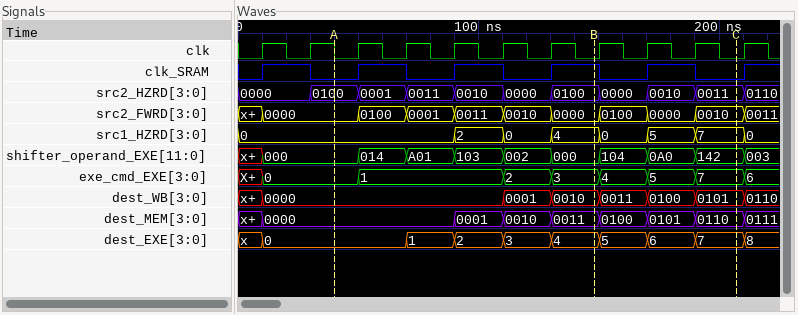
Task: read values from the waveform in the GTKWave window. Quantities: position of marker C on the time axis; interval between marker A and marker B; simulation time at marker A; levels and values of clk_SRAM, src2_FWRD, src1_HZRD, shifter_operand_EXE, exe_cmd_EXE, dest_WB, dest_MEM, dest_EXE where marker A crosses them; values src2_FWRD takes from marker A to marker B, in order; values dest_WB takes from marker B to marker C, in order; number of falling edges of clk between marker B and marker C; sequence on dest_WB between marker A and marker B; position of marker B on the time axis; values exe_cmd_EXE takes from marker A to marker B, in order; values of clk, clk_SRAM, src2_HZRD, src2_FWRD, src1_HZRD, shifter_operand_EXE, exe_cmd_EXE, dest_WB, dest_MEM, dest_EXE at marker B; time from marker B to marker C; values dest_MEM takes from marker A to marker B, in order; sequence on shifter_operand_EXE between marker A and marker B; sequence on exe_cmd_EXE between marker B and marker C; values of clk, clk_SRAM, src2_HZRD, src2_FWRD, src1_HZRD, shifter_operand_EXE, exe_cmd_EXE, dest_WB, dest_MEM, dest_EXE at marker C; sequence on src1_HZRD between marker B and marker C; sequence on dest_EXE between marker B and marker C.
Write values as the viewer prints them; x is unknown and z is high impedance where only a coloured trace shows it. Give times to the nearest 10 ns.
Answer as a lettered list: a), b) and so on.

a) 210 ns
b) 110 ns
c) 40 ns
d) clk_SRAM=0, src2_FWRD=0000, src1_HZRD=0, shifter_operand_EXE=000, exe_cmd_EXE=0, dest_WB=0000, dest_MEM=0000, dest_EXE=0
e) 0000, 0100, 0001, 0011, 0010, 0000
f) 0010, 0011, 0100, 0101
g) 3
h) 0000, 0001, 0010
i) 150 ns
j) 0, 1, 2, 3
k) clk=0, clk_SRAM=1, src2_HZRD=0100, src2_FWRD=0000, src1_HZRD=4, shifter_operand_EXE=000, exe_cmd_EXE=3, dest_WB=0010, dest_MEM=0011, dest_EXE=4
l) 60 ns
m) 0000, 0001, 0010, 0011
n) 000, 014, A01, 103, 002, 000
o) 3, 4, 5, 7
p) clk=0, clk_SRAM=0, src2_HZRD=0011, src2_FWRD=0010, src1_HZRD=7, shifter_operand_EXE=142, exe_cmd_EXE=7, dest_WB=0101, dest_MEM=0110, dest_EXE=7
q) 4, 0, 5, 7
r) 4, 5, 6, 7
